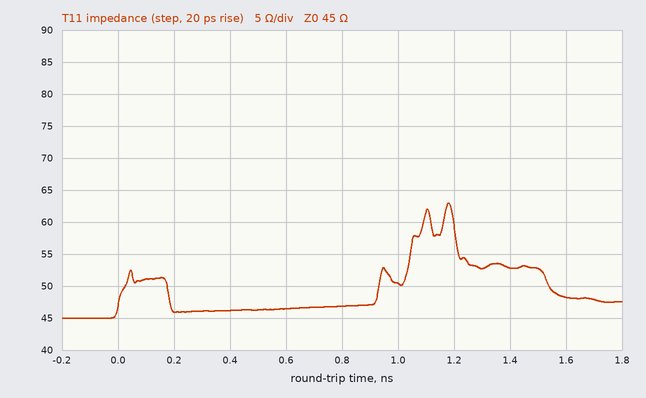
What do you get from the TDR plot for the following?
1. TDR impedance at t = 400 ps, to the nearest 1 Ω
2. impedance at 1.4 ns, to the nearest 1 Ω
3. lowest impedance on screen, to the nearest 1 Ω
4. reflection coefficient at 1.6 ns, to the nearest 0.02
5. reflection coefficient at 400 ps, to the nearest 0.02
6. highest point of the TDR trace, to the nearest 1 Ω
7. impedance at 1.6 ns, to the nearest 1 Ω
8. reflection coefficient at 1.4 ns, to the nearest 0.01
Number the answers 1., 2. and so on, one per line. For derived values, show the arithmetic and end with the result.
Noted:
1. 46 Ω
2. 53 Ω
3. 45 Ω
4. (48 − 45)/(48 + 45) ≈ +0.0323, so +0.04 to the nearest 0.02
5. (46 − 45)/(46 + 45) ≈ +0.0110, so +0.02 to the nearest 0.02
6. 63 Ω
7. 48 Ω
8. (53 − 45)/(53 + 45) ≈ +0.08
